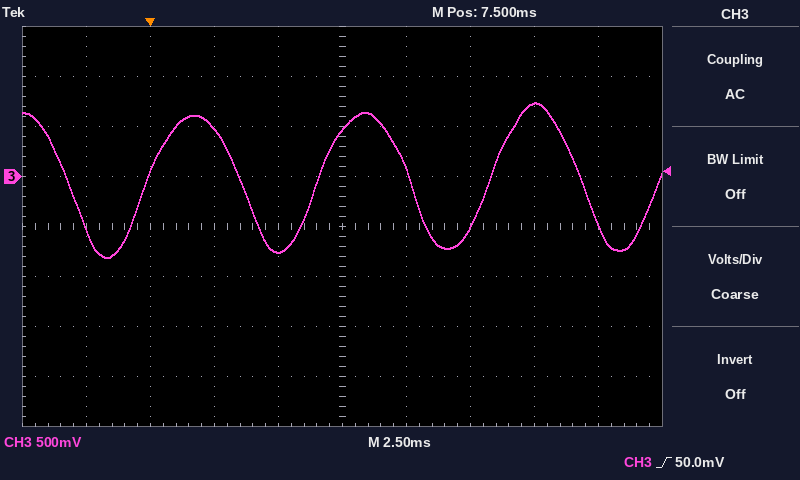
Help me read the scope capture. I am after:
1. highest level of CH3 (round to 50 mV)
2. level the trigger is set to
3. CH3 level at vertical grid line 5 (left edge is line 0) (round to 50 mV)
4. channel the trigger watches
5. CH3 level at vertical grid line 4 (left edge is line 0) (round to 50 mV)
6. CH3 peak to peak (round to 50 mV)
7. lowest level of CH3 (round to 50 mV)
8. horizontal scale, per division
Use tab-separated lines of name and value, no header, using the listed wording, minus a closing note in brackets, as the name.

highest level of CH3	750 mV
level the trigger is set to	50.0 mV
CH3 level at vertical grid line 5 (left edge is line 0)	450 mV
channel the trigger watches	CH3
CH3 level at vertical grid line 4 (left edge is line 0)	-750 mV
CH3 peak to peak	1.55 V
lowest level of CH3	-800 mV
horizontal scale, per division	2.5 ms
